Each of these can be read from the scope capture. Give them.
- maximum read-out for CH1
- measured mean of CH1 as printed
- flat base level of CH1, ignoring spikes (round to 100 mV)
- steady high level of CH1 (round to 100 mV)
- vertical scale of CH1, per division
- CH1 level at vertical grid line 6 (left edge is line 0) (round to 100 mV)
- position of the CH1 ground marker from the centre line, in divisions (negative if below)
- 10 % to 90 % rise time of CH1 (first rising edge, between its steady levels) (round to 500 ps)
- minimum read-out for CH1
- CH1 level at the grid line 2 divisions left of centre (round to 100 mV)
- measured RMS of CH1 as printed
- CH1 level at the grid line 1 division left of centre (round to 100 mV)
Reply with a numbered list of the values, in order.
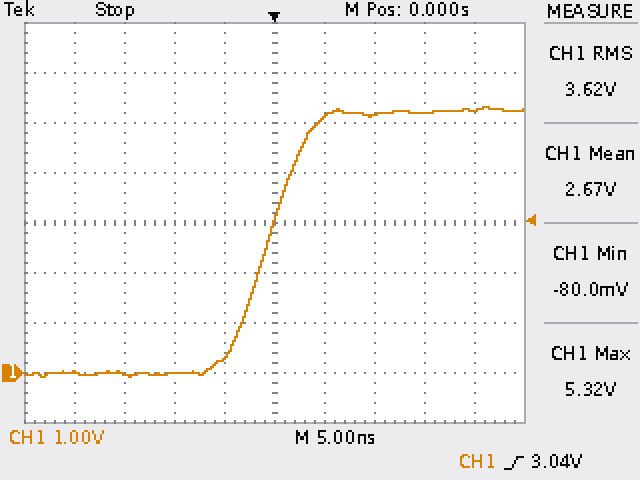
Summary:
1. 5.32 V
2. 2.67 V
3. 0.0 V
4. 5.2 V
5. 1 V
6. 5.1 V
7. -3.0 div
8. 7.5 ns
9. -80.0 mV
10. 0.0 V
11. 3.62 V
12. 300 mV
